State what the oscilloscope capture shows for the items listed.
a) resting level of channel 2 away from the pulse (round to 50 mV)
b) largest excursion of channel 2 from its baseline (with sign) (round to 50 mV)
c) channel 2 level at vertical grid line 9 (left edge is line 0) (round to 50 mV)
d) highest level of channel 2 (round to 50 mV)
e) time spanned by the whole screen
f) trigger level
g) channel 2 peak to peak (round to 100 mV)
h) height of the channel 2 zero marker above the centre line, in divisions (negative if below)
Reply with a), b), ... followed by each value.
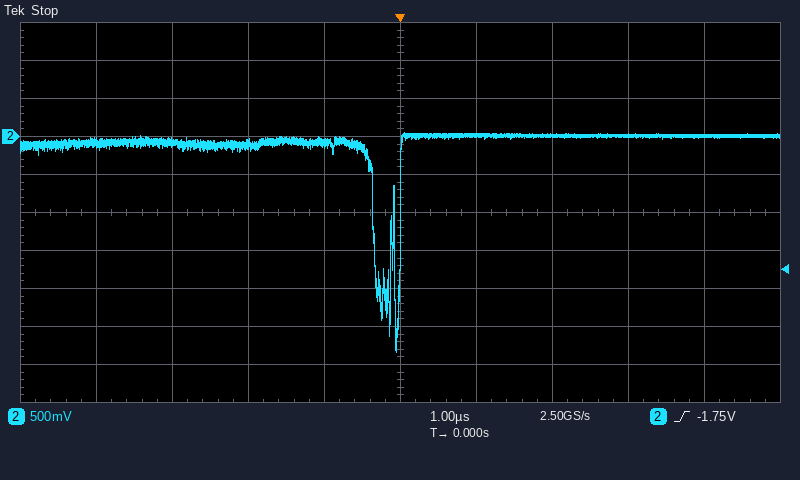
a) 0 mV
b) -2.85 V
c) 0 mV
d) 50 mV
e) 10 µs
f) -1.75 V
g) 2.90 V
h) +2.0 div
